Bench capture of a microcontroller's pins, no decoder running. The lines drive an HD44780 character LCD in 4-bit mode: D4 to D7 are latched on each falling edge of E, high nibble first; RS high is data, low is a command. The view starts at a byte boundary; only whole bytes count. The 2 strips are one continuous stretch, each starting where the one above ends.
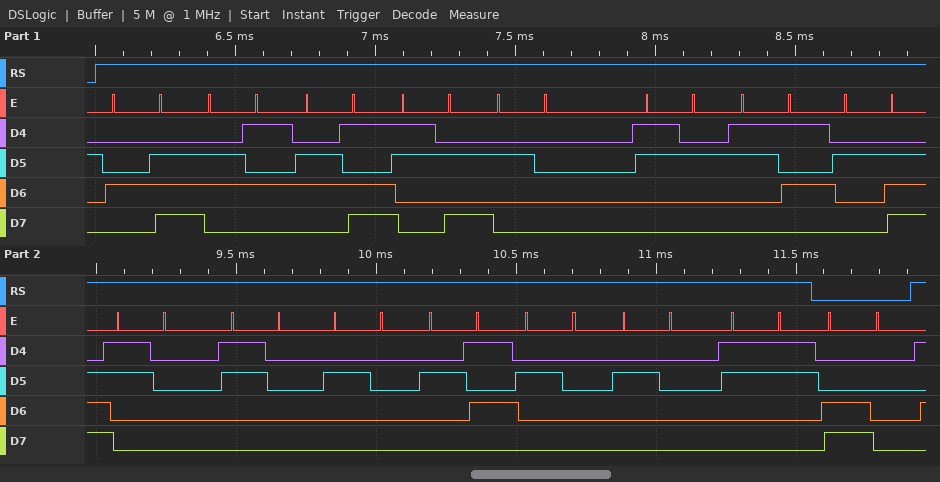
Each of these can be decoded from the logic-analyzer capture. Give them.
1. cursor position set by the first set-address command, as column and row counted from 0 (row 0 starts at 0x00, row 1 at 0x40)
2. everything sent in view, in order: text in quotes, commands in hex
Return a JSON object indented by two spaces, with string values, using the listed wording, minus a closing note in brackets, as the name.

{
  "cursor position set by the first set-address command, as column and row counted from 0": "column 0, row 1",
  "everything sent in view, in order: text in quotes, commands in hex": "\"Nem: 25.00 %  3\" 0xC0"
}
